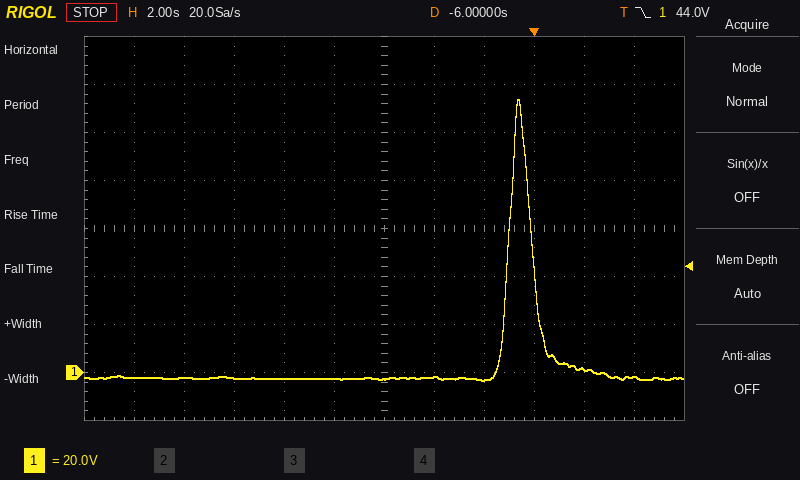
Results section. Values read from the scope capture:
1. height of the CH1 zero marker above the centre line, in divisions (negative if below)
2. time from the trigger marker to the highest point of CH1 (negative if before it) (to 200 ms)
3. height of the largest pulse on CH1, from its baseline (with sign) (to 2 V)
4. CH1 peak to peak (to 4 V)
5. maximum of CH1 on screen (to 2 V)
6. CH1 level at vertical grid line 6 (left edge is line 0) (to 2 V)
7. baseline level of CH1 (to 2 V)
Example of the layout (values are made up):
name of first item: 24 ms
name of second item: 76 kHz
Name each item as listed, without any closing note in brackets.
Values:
height of the CH1 zero marker above the centre line, in divisions: -3.0 div
time from the trigger marker to the highest point of CH1 (negative if before it): -600 ms
height of the largest pulse on CH1, from its baseline (with sign): +116 V
CH1 peak to peak: 116 V
maximum of CH1 on screen: 114 V
CH1 level at vertical grid line 6 (left edge is line 0): -2 V
baseline level of CH1: -2 V
